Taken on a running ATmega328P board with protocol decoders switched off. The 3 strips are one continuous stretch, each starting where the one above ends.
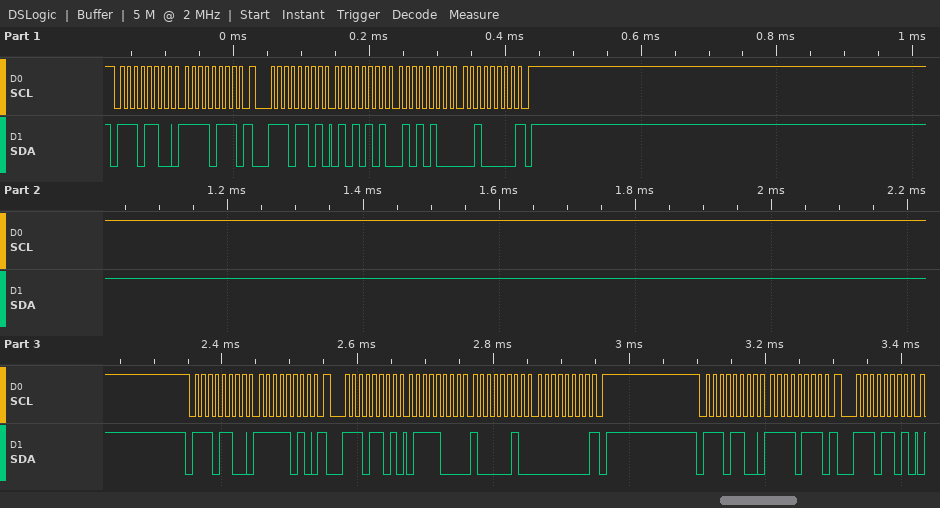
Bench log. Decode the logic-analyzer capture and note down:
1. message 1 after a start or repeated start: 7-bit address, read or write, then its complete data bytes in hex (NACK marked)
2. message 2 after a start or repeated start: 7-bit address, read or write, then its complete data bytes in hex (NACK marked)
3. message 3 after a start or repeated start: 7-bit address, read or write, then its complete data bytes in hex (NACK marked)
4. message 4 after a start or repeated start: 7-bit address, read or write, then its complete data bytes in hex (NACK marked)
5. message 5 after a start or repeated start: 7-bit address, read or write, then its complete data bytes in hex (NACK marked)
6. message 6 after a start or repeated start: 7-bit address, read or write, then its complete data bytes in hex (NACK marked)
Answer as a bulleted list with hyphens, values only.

- 0x76 write: F7
- 0x76 read: 55 54 20 NACK
- 0x76 write: FA
- 0x76 read: 78 82 00 NACK
- 0x76 write: F7
- 0x76 read
